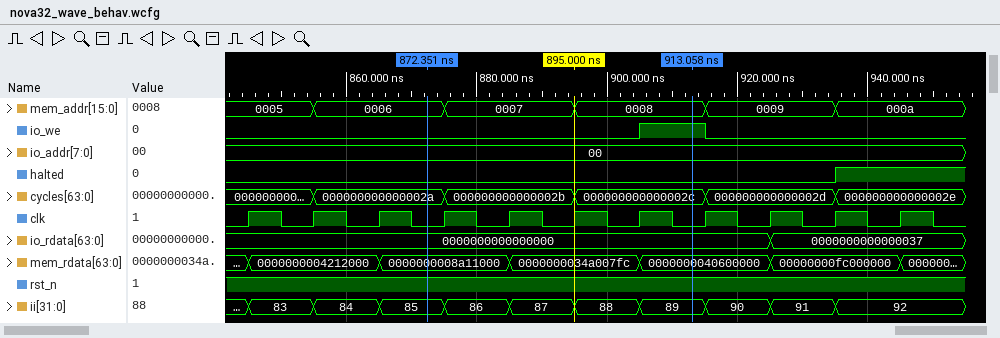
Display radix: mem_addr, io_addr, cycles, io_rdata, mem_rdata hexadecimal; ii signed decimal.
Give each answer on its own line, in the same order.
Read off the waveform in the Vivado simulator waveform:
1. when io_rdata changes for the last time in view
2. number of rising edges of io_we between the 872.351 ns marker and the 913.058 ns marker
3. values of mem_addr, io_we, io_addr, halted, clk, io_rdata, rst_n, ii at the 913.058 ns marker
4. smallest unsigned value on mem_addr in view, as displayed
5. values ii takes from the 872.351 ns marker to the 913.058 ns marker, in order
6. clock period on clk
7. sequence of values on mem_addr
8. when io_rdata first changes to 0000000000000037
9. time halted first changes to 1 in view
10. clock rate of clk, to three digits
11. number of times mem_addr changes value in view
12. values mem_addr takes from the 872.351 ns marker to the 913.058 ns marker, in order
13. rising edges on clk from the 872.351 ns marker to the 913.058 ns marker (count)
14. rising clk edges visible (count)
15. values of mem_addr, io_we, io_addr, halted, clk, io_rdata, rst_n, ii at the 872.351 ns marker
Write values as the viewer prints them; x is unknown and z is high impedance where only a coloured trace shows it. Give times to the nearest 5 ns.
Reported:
925 ns
1
mem_addr=0008, io_we=1, io_addr=00, halted=0, clk=0, io_rdata=0000000000000000, rst_n=1, ii=89
0005
85, 86, 87, 88, 89
10 ns
0005, 0006, 0007, 0008, 0009, 000a
925 ns
935 ns
100 MHz
5
0006, 0007, 0008
4
11
mem_addr=0006, io_we=0, io_addr=00, halted=0, clk=0, io_rdata=0000000000000000, rst_n=1, ii=85
